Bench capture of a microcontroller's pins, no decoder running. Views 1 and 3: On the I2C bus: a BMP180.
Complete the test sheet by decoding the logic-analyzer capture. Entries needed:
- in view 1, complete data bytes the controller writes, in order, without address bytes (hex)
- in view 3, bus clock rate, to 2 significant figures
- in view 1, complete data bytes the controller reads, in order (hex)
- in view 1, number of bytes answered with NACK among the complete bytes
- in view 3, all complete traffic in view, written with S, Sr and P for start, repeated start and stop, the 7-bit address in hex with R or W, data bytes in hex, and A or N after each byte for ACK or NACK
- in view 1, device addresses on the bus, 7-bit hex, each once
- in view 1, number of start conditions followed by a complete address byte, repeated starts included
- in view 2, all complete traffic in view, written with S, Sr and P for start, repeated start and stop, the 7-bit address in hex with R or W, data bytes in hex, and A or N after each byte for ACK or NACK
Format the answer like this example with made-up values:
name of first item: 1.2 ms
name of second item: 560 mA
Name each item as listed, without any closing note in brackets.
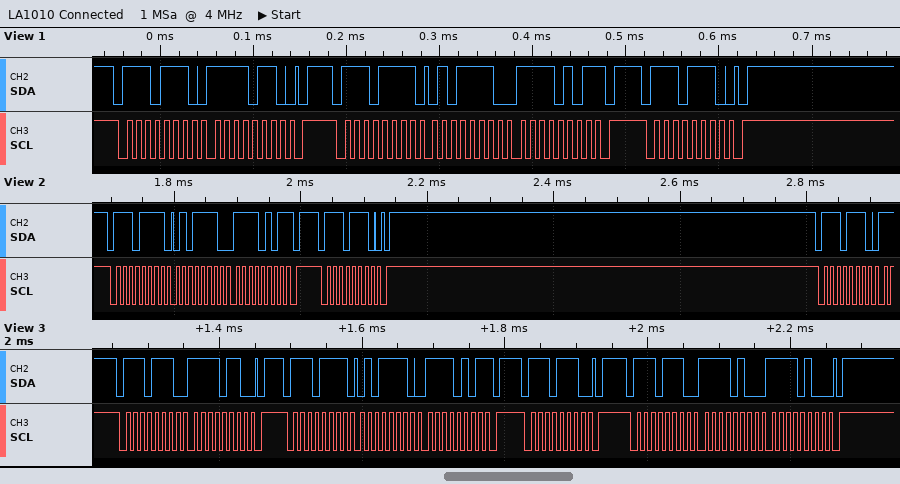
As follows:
in view 1, complete data bytes the controller writes, in order, without address bytes: F6
in view 3, bus clock rate, to 2 significant figures: 100 kHz
in view 1, complete data bytes the controller reads, in order: 5E F5
in view 1, number of bytes answered with NACK among the complete bytes: 1
in view 3, all complete traffic in view, written with S, Sr and P for start, repeated start and stop, the 7-bit address in hex with R or W, data bytes in hex, and A or N after each byte for ACK or NACK: S 77W A F6 A P S 77R A 5E A F5 N P S 77W A P S 77W A F4 A F4 A P
in view 1, device addresses on the bus, 7-bit hex, each once: 0x77
in view 1, number of start conditions followed by a complete address byte, repeated starts included: 3
in view 2, all complete traffic in view, written with S, Sr and P for start, repeated start and stop, the 7-bit address in hex with R or W, data bytes in hex, and A or N after each byte for ACK or NACK: S 77R A 5E A F5 N P S 77W A P S 77W A
